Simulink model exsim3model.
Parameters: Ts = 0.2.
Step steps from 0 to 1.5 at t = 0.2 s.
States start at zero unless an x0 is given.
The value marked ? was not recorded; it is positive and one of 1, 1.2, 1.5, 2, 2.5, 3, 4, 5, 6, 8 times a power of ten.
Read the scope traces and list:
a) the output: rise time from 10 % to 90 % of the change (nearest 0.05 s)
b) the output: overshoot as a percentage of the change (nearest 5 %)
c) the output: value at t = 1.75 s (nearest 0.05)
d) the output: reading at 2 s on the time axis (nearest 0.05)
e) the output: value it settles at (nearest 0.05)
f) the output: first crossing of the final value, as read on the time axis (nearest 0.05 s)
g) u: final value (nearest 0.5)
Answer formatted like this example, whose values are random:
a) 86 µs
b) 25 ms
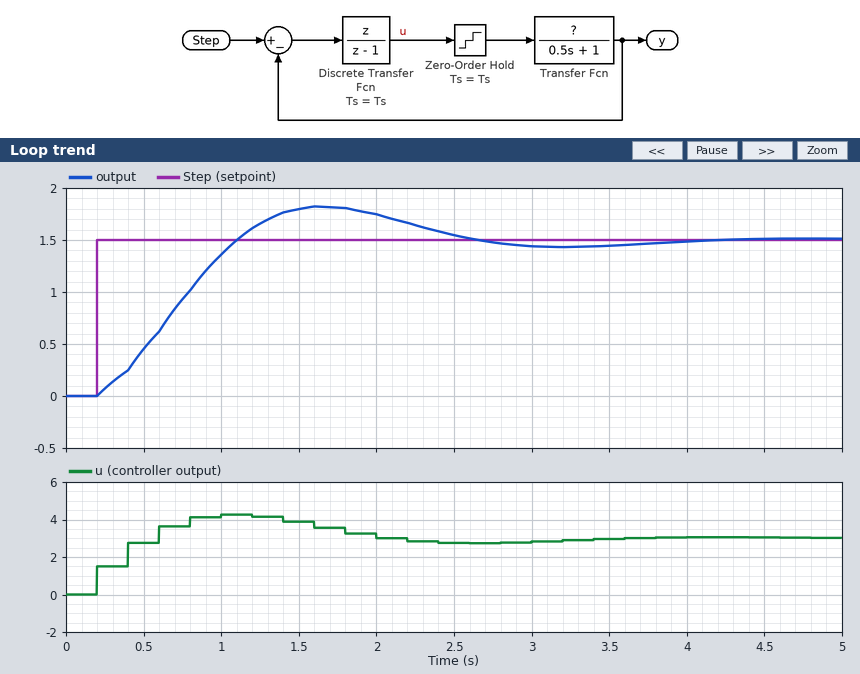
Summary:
a) 0.70 s
b) 20 %
c) 1.80
d) 1.75
e) 1.50
f) 1.10 s
g) 3.0
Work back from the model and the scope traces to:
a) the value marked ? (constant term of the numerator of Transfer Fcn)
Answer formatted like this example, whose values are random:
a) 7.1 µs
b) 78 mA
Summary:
a) 0.5
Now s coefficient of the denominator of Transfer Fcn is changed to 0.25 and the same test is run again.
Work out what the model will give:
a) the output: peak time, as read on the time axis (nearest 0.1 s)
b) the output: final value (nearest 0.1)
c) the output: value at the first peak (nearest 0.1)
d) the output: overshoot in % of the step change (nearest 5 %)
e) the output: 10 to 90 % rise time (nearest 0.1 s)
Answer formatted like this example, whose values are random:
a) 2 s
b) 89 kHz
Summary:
a) 1.4 s
b) 1.5
c) 1.6
d) 10 %
e) 0.6 s
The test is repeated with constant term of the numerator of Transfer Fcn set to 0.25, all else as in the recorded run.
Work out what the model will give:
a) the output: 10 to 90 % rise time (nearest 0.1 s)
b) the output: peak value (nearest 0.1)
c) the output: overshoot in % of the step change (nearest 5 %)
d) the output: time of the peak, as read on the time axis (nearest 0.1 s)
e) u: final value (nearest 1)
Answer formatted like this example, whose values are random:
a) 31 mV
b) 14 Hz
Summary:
a) 1.2 s
b) 1.6
c) 10 %
d) 2.6 s
e) 6
